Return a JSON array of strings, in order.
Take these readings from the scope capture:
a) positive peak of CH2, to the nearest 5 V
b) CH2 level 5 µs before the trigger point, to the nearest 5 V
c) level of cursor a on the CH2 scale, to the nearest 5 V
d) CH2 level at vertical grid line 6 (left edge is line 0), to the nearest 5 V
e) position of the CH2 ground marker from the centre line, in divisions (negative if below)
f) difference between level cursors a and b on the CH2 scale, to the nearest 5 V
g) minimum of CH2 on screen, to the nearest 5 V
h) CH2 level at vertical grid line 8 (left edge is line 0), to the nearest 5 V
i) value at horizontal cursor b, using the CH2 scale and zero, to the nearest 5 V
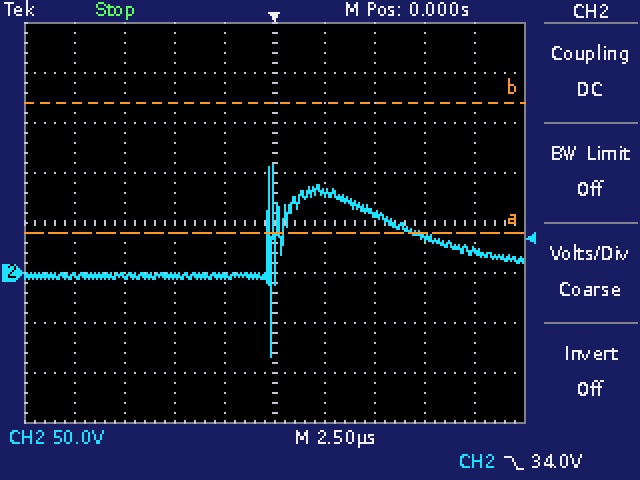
["110 V", "-5 V", "40 V", "80 V", "-1.0 div", "130 V", "-85 V", "35 V", "170 V"]
